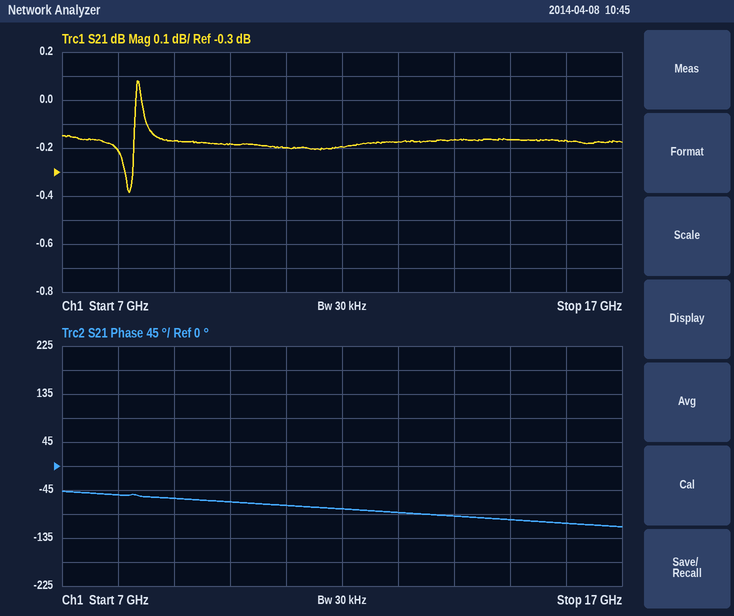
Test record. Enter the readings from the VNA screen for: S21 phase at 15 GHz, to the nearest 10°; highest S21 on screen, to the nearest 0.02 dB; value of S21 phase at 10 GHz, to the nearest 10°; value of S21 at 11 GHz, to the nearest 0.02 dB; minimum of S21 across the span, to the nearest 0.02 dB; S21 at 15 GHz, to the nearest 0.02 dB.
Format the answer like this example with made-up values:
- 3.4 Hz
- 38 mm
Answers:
- -100°
- 0.08 dB
- -70°
- -0.20 dB
- -0.38 dB
- -0.16 dB
